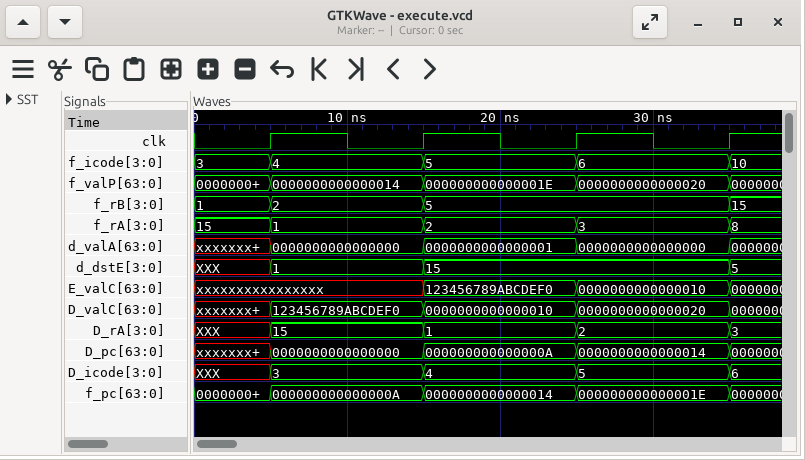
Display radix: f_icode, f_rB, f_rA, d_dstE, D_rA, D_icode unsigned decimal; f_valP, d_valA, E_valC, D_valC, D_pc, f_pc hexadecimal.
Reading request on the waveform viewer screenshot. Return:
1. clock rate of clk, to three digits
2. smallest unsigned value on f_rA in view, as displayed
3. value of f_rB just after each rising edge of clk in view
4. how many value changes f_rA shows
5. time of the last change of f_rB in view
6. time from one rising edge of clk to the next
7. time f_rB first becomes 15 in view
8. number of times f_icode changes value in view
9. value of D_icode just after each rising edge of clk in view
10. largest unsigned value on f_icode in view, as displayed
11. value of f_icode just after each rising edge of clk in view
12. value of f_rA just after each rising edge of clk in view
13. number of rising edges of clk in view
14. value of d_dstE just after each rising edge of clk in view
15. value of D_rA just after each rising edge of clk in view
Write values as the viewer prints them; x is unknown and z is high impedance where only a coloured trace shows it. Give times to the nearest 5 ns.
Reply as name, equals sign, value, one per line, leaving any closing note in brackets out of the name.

clock rate of clk, to three digits = 100 MHz
smallest unsigned value on f_rA in view, as displayed = 1
value of f_rB just after each rising edge of clk in view = 2, 5, 5, 15
how many value changes f_rA shows = 4
time of the last change of f_rB in view = 35 ns
time from one rising edge of clk to the next = 10 ns
time f_rB first becomes 15 in view = 35 ns
number of times f_icode changes value in view = 4
value of D_icode just after each rising edge of clk in view = 3, 4, 5, 6
largest unsigned value on f_icode in view, as displayed = 10
value of f_icode just after each rising edge of clk in view = 4, 5, 6, 10
value of f_rA just after each rising edge of clk in view = 1, 2, 3, 8
number of rising edges of clk in view = 4
value of d_dstE just after each rising edge of clk in view = 1, 15, 15, 5
value of D_rA just after each rising edge of clk in view = 15, 1, 2, 3
